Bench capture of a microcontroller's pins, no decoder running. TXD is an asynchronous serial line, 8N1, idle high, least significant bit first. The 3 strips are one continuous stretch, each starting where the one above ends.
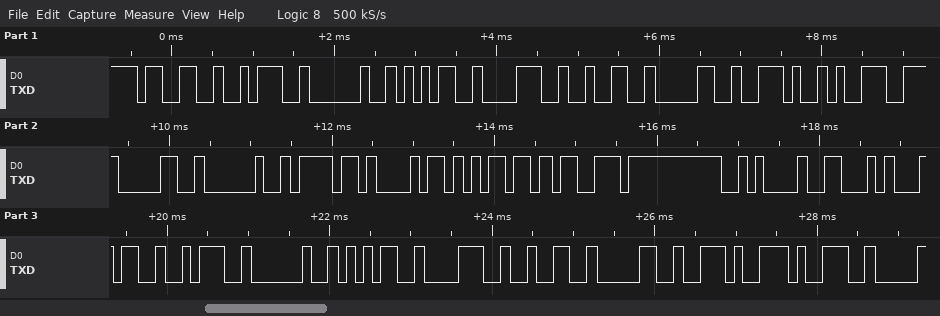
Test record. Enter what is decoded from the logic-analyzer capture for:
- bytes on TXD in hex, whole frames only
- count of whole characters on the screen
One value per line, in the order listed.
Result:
33 3A 20 35 38 32 30 2E 39 30 20 6F 68 6D 73 0A 46 34 3A 20 35 38 32 30 2E 39
26
